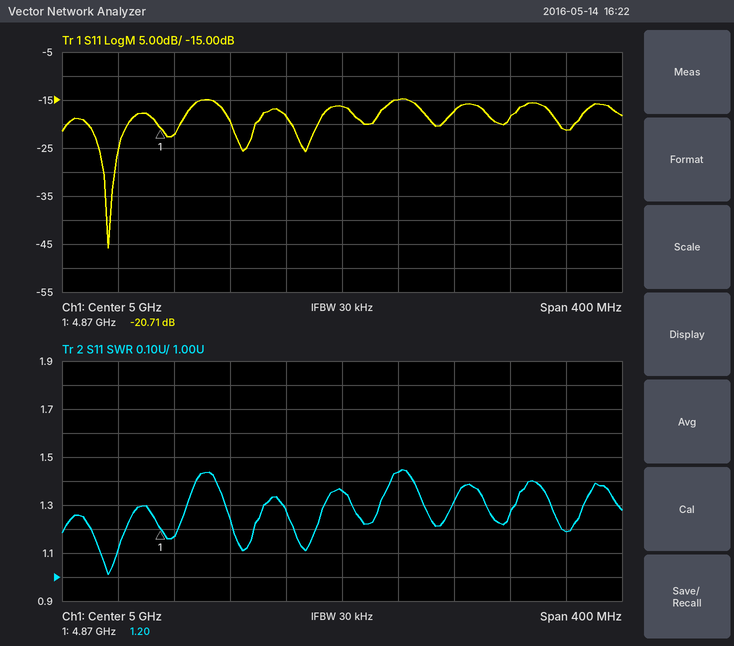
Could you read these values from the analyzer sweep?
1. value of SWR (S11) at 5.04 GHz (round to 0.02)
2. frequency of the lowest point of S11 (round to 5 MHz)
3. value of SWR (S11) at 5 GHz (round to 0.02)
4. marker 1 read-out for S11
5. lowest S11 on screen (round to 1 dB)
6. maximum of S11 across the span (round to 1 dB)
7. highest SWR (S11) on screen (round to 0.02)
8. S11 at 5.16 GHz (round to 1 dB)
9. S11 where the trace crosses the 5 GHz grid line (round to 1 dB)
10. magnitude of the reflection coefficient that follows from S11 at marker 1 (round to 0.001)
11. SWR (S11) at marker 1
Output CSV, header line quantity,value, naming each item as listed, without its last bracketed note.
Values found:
quantity,value
value of SWR (S11) at 5.04 GHz,1.44
frequency of the lowest point of S11,4.835 GHz
value of SWR (S11) at 5 GHz,1.36
marker 1 read-out for S11,-20.71 dB
lowest S11 on screen,-46 dB
maximum of S11 across the span,-15 dB
highest SWR (S11) on screen,1.44
S11 at 5.16 GHz,-21 dB
S11 where the trace crosses the 5 GHz grid line,-16 dB
magnitude of the reflection coefficient that follows from S11 at marker 1,0.092
SWR (S11) at marker 1,1.20
